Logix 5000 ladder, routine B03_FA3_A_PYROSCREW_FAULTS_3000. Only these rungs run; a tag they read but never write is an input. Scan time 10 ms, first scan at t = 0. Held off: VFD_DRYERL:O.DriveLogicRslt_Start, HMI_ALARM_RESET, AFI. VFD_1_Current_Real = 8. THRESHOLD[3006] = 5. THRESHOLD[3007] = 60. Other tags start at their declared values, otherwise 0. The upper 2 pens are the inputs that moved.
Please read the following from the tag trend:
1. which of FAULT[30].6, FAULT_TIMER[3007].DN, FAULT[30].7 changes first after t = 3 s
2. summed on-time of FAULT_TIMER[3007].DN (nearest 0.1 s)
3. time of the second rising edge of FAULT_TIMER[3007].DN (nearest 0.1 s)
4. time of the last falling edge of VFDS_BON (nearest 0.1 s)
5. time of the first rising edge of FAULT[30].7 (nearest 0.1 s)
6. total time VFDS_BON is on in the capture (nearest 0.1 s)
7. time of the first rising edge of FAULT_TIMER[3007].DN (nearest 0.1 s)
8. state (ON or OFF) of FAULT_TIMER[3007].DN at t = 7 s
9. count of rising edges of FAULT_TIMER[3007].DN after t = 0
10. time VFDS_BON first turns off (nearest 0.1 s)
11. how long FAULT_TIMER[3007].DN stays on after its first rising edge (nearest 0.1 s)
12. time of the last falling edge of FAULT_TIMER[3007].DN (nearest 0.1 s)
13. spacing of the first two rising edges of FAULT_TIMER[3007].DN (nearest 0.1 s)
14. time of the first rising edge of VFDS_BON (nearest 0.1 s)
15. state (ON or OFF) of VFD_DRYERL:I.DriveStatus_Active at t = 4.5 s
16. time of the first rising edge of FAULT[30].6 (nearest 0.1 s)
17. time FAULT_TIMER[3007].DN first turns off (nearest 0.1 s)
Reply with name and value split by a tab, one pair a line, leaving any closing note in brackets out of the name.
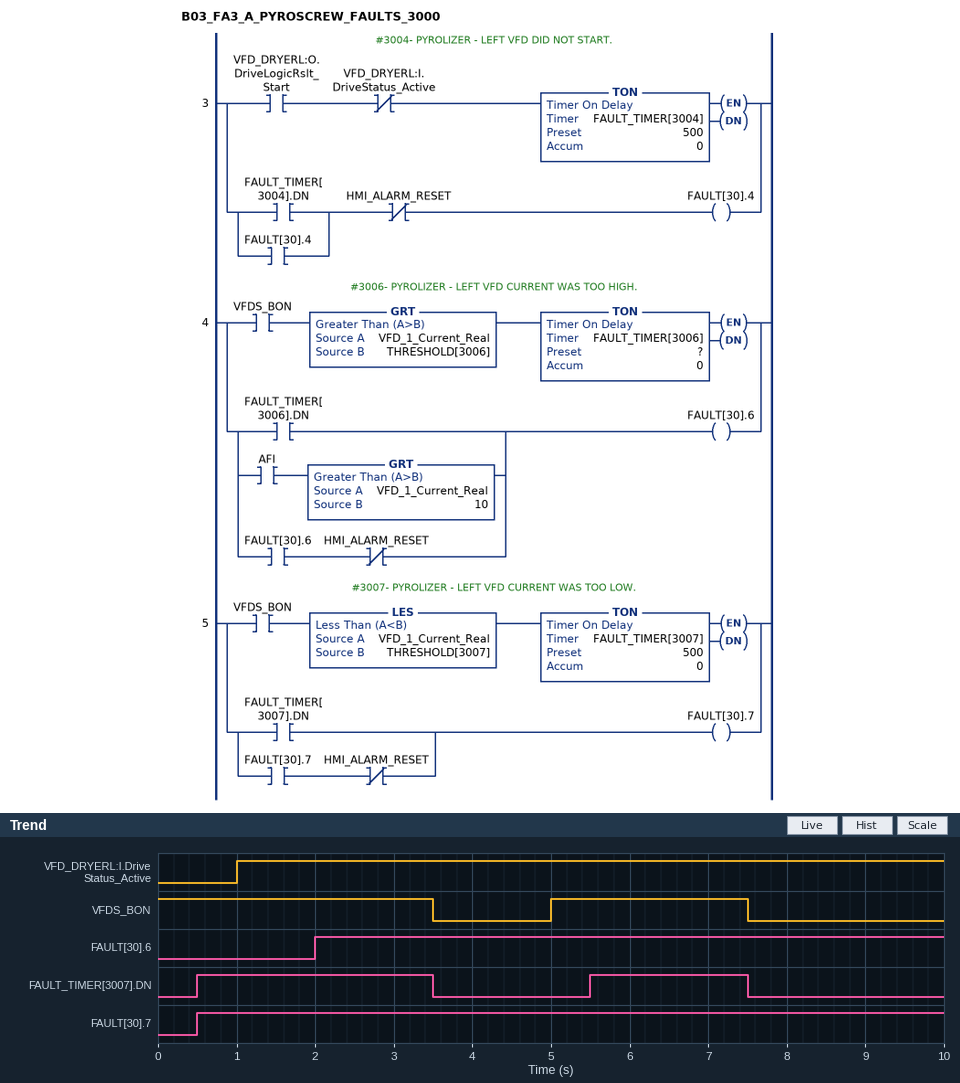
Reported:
which of FAULT[30].6, FAULT_TIMER[3007].DN, FAULT[30].7 changes first after t = 3 s	FAULT_TIMER[3007].DN
summed on-time of FAULT_TIMER[3007].DN	5.0 s
time of the second rising edge of FAULT_TIMER[3007].DN	5.5 s
time of the last falling edge of VFDS_BON	7.5 s
time of the first rising edge of FAULT[30].7	0.5 s
total time VFDS_BON is on in the capture	6.0 s
time of the first rising edge of FAULT_TIMER[3007].DN	0.5 s
state (ON or OFF) of FAULT_TIMER[3007].DN at t = 7 s	ON
count of rising edges of FAULT_TIMER[3007].DN after t = 0	2
time VFDS_BON first turns off	3.5 s
how long FAULT_TIMER[3007].DN stays on after its first rising edge	3.0 s
time of the last falling edge of FAULT_TIMER[3007].DN	7.5 s
spacing of the first two rising edges of FAULT_TIMER[3007].DN	5.0 s
time of the first rising edge of VFDS_BON	5.0 s
state (ON or OFF) of VFD_DRYERL:I.DriveStatus_Active at t = 4.5 s	ON
time of the first rising edge of FAULT[30].6	2.0 s
time FAULT_TIMER[3007].DN first turns off	3.5 s
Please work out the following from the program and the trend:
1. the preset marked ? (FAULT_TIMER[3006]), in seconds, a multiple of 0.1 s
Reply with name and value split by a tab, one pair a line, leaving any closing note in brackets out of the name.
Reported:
the preset marked ? (FAULT_TIMER[3006]), in seconds, a multiple of 0.1 s	2.0 s
